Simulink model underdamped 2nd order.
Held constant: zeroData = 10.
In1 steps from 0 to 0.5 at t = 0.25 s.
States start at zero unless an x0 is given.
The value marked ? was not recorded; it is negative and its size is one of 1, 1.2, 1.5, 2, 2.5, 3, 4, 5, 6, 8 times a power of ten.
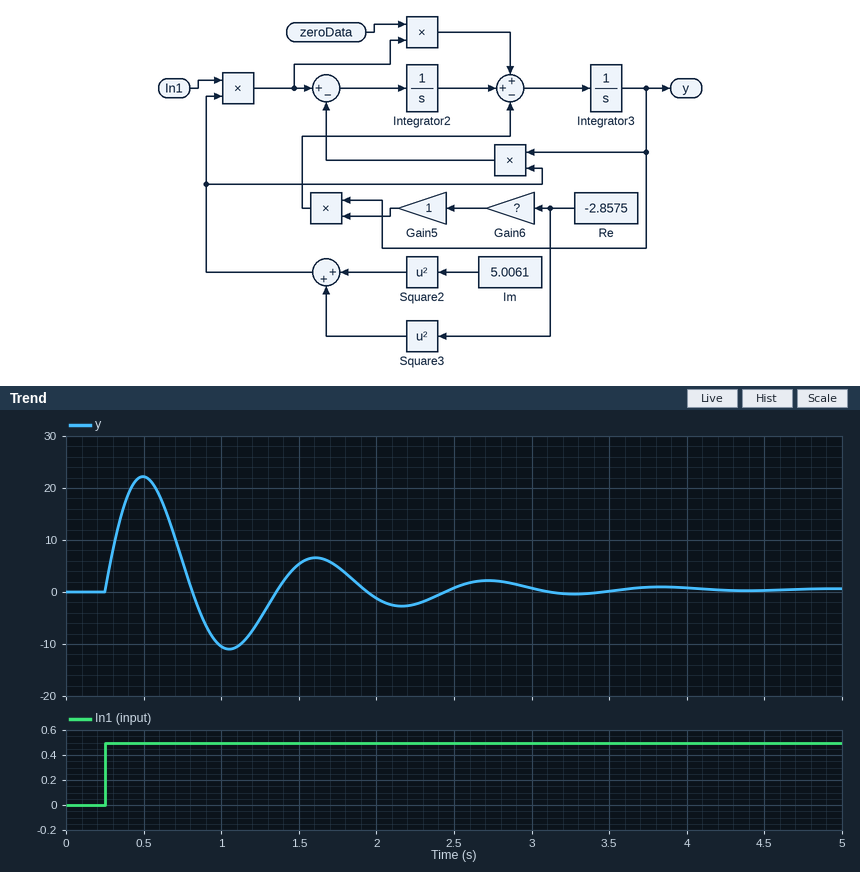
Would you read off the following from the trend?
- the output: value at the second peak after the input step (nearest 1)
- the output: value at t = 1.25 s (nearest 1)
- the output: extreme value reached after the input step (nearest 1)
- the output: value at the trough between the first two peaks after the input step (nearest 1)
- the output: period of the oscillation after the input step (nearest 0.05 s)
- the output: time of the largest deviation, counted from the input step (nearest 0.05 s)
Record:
7
-5
22
-11
1.10 s
0.25 s
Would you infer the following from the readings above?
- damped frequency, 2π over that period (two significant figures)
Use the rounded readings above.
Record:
5.7 rad/s
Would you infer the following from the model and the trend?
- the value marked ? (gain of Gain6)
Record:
-0.8
